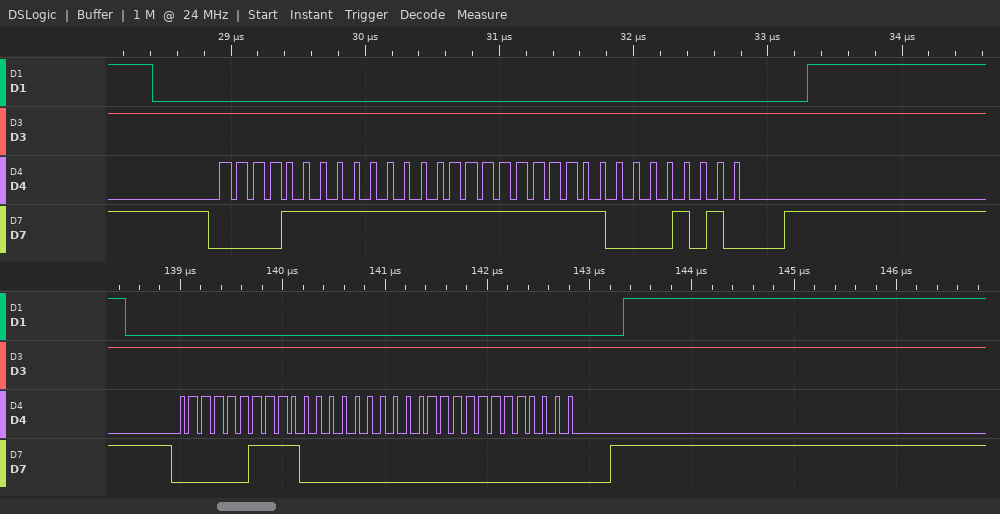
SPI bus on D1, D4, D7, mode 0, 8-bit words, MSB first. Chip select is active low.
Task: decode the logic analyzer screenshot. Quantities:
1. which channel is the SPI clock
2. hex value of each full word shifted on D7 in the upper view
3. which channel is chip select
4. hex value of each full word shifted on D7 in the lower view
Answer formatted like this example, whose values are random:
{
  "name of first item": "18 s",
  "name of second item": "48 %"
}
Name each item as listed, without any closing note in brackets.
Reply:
{
  "which channel is the SPI clock": "D4",
  "hex value of each full word shifted on D7 in the upper view": "0F, FF, FF, 0A",
  "which channel is chip select": "D1",
  "hex value of each full word shifted on D7 in the lower view": "03, C0, 00, 00"
}
